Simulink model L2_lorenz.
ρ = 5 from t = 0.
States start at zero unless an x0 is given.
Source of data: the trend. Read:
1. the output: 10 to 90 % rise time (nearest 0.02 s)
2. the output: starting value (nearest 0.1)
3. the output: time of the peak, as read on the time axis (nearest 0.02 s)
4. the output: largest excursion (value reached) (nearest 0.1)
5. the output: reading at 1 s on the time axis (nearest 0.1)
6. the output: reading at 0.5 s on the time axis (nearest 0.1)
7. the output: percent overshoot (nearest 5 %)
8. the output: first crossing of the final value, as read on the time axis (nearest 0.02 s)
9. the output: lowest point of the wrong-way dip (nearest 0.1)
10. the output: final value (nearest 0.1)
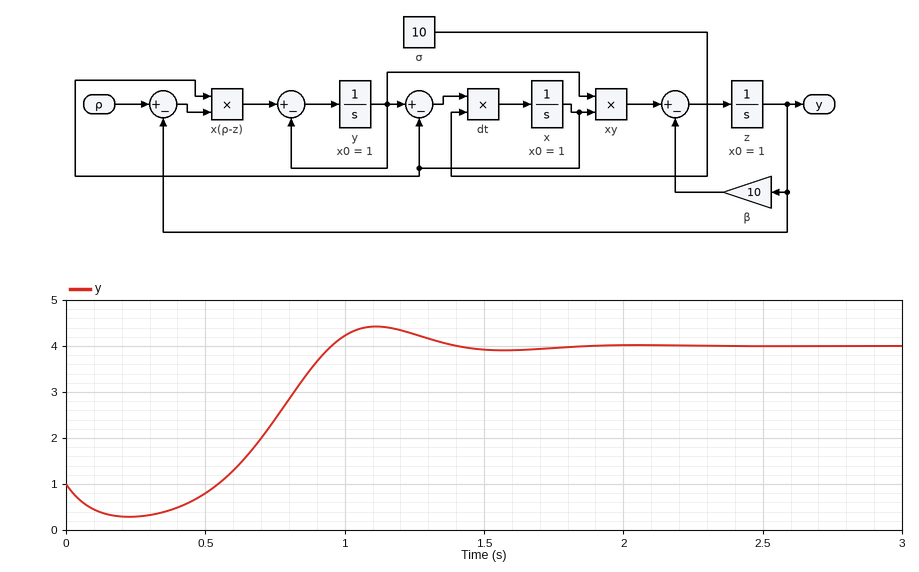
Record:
0.30 s
1.0
1.12 s
4.4
4.2
0.8
15 %
0.96 s
0.3
4.0
